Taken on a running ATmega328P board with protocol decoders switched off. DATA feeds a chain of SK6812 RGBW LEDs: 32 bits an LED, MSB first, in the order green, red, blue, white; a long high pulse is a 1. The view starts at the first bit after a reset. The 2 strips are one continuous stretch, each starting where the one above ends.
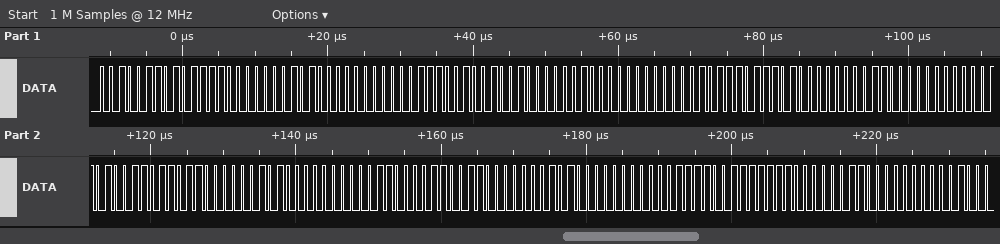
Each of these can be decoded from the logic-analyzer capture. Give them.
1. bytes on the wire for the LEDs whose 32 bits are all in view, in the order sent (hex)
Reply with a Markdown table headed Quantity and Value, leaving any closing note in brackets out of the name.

| Quantity | Value |
|---|---|
| bytes on the wire for the LEDs whose 32 bits are all in view, in the order sent | 26 BC 05 00 1C 92 04 00 2E E8 06 00 29 B6 05 00 30 CC 05 00 1E 7F 03 00 |
